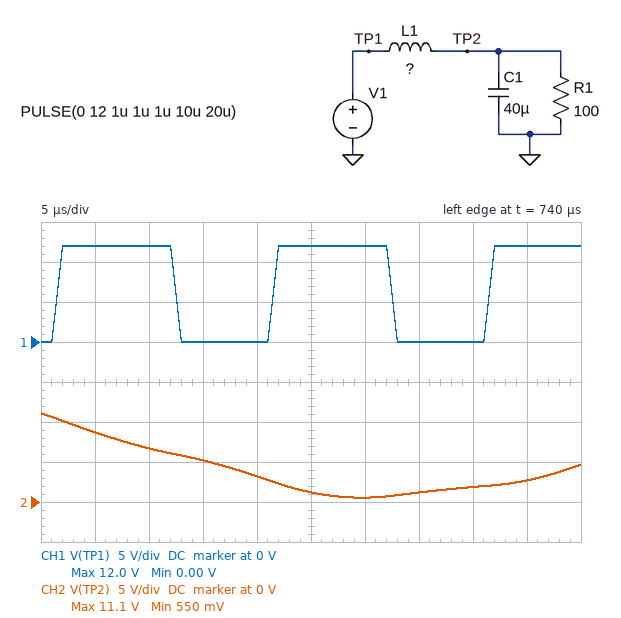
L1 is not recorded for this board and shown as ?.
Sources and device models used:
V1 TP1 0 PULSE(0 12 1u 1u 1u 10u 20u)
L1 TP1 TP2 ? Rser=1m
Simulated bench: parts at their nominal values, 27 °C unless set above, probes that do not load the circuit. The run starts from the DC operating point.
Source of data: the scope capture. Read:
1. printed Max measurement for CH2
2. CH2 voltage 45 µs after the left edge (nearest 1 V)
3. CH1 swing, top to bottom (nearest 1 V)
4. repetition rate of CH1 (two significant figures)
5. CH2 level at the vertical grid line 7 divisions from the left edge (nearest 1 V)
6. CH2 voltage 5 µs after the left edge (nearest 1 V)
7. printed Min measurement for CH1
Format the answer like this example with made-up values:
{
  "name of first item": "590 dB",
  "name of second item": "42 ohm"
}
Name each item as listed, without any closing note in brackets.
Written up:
{
  "printed Max measurement for CH2": "11.1 V",
  "CH2 voltage 45 µs after the left edge": "3 V",
  "CH1 swing, top to bottom": "12 V",
  "repetition rate of CH1": "50 kHz",
  "CH2 level at the vertical grid line 7 divisions from the left edge": "1 V",
  "CH2 voltage 5 µs after the left edge": "9 V",
  "printed Min measurement for CH1": "0.00 V"
}
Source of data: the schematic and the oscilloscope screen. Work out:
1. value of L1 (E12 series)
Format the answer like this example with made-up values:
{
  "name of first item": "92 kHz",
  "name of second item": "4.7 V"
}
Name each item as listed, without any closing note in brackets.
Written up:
{
  "value of L1": "4.7 µH"
}
